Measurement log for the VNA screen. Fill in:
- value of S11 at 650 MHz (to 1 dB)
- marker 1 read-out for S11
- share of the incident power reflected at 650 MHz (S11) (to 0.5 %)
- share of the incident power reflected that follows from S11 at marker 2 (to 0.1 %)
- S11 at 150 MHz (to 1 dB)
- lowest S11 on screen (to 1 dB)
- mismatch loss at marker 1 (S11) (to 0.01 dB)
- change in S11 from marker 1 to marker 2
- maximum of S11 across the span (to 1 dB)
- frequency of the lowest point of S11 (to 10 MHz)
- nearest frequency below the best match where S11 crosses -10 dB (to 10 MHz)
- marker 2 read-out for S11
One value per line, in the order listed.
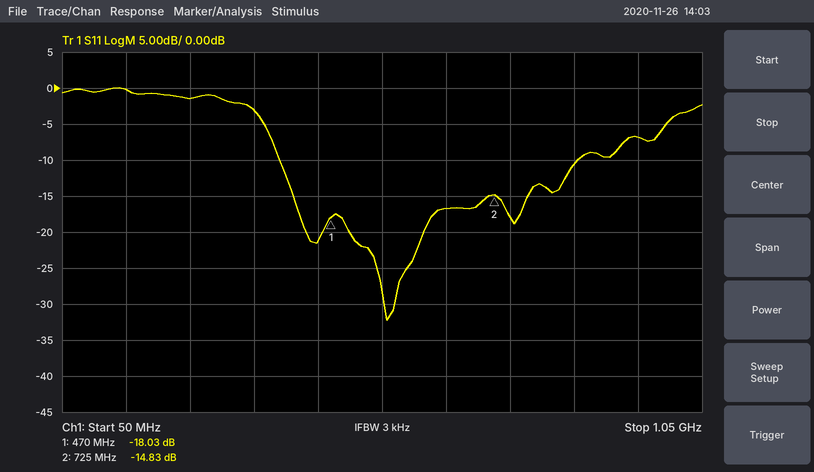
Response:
-17 dB
-18.03 dB
2.0 %
3.3 %
0 dB
-32 dB
0.07 dB
3.20 dB
0 dB
560 MHz
390 MHz
-14.83 dB
